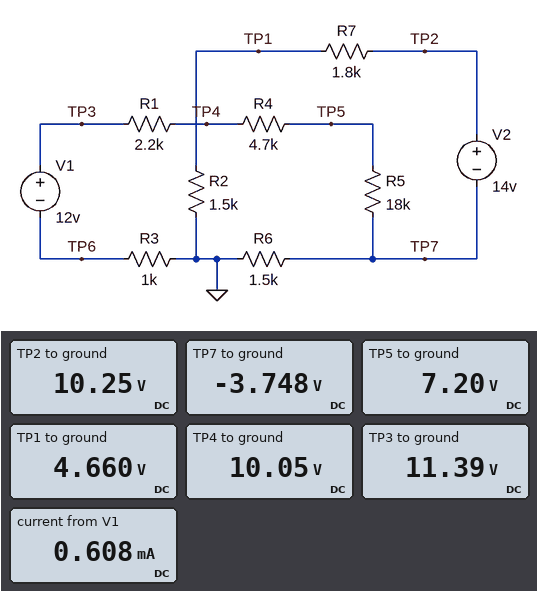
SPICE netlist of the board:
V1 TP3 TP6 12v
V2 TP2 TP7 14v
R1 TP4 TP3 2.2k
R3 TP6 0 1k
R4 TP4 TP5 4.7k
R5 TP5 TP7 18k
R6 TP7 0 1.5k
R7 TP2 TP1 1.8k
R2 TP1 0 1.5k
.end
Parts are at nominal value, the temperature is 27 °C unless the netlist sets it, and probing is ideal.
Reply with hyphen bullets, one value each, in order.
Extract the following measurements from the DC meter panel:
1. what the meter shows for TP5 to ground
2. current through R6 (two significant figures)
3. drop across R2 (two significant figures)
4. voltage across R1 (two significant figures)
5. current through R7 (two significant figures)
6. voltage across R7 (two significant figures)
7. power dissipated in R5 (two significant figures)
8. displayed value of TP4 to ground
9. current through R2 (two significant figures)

- 7.20 V
- 2.5 mA
- 4.7 V
- 1.3 V
- 3.1 mA
- 5.6 V
- 6.7 mW
- 10.05 V
- 3.1 mA
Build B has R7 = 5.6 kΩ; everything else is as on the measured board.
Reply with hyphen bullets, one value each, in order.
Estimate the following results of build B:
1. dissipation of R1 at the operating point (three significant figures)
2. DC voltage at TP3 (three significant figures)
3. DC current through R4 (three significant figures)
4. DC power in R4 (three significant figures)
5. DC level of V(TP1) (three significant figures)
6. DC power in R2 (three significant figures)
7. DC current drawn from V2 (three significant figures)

- 623 µW
- 11.5 V
- 532 µA
- 1.33 mW
- 2.58 V
- 4.44 mW
- 1.72 mA
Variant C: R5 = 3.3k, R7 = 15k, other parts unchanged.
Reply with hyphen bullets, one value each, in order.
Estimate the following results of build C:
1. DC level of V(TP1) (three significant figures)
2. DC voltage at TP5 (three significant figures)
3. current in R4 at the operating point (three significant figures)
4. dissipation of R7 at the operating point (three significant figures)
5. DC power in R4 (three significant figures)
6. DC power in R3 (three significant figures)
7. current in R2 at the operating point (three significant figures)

- 1.30 V
- 3.73 V
- 1.05 mA
- 11.2 mW
- 5.15 mW
- 1.10 mW
- 865 µA
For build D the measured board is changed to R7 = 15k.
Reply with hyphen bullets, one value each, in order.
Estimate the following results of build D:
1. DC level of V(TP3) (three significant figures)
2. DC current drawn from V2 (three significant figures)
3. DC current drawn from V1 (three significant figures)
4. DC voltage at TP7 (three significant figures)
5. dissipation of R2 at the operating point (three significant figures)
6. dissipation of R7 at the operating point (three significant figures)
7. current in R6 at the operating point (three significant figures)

- 11.5 V
- 818 µA
- 483 µA
- -503 mV
- 1.00 mW
- 10.0 mW
- 335 µA
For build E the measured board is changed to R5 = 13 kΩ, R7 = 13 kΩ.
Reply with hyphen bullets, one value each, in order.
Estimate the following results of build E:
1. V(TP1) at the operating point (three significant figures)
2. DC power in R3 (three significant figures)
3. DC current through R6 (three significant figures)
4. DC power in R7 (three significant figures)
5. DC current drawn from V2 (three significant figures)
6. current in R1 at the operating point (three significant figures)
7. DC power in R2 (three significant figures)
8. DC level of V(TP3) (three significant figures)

- 1.40 V
- 358 µW
- 333 µA
- 11.3 mW
- 931 µA
- 598 µA
- 1.30 mW
- 11.4 V
